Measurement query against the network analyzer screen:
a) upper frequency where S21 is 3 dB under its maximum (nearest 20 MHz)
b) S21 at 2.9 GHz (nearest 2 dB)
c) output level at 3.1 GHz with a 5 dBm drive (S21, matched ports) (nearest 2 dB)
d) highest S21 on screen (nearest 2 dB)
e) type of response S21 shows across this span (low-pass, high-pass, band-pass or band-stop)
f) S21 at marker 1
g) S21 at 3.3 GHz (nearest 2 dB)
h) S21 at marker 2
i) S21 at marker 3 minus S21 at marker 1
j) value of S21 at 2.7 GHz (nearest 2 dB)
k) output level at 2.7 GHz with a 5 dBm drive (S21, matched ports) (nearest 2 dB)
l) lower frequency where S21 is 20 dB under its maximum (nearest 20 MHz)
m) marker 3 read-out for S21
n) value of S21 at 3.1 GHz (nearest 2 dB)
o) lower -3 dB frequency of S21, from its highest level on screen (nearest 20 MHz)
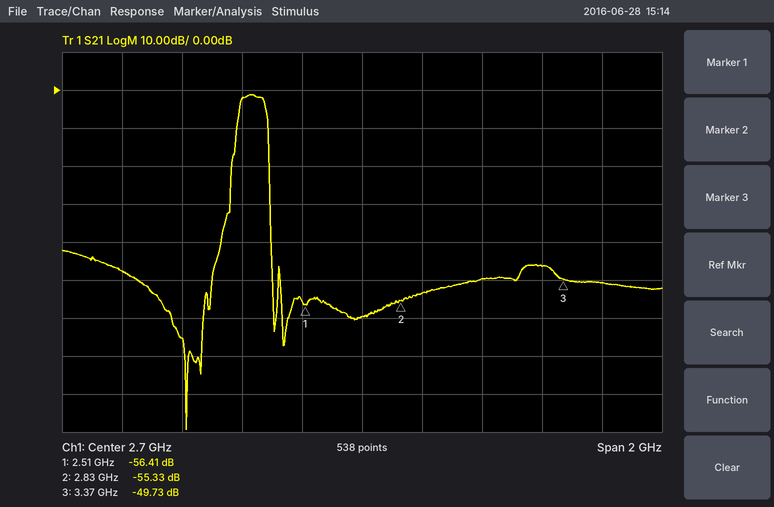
2.38 GHz
-54 dB
-44 dBm
-2 dB
band-pass
-56.41 dB
-46 dB
-55.33 dB
6.68 dB
-60 dB
-54 dBm
2.26 GHz
-49.73 dB
-50 dB
2.30 GHz
